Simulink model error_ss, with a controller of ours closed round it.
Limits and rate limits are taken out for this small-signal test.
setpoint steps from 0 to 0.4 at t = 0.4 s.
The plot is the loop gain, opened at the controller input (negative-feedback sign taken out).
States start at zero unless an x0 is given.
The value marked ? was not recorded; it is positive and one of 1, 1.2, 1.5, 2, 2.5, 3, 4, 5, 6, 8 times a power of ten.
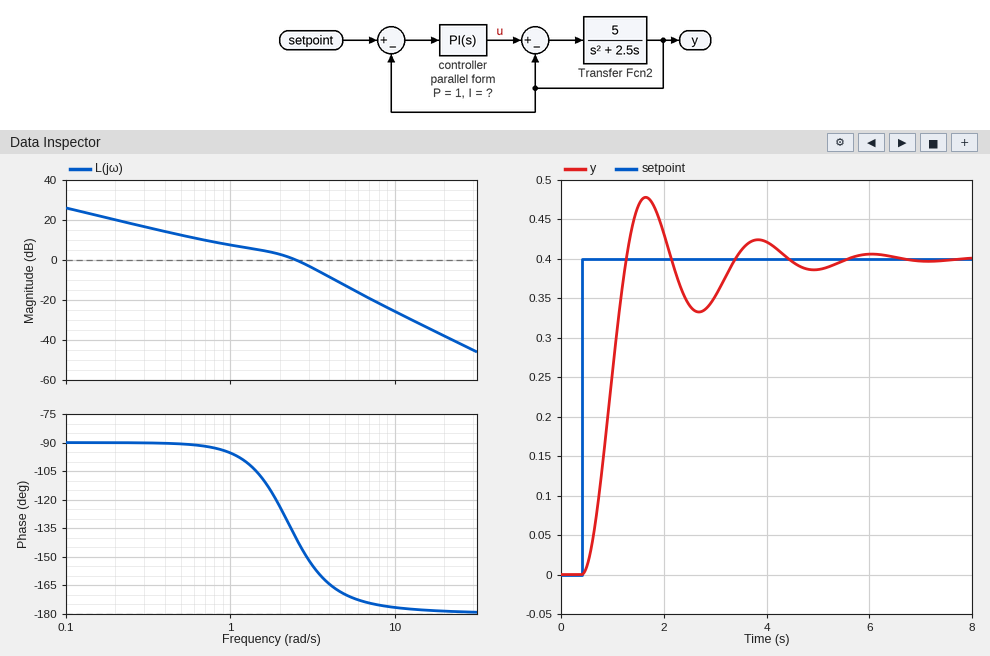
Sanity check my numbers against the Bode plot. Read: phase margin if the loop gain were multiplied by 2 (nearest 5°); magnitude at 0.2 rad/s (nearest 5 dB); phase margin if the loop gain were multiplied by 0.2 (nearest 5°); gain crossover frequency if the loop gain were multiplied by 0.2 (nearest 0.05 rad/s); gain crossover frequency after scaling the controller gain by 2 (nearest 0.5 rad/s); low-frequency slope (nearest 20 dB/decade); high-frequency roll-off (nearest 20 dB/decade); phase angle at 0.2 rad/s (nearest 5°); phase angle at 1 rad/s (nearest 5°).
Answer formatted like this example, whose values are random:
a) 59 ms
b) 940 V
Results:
a) 20°
b) 20 dB
c) 90°
d) 0.40 rad/s
e) 3.5 rad/s
f) -20 dB/decade
g) -40 dB/decade
h) -90°
i) -95°
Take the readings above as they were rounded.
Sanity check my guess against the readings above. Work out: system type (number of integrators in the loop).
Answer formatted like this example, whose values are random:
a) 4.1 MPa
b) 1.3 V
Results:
a) 1
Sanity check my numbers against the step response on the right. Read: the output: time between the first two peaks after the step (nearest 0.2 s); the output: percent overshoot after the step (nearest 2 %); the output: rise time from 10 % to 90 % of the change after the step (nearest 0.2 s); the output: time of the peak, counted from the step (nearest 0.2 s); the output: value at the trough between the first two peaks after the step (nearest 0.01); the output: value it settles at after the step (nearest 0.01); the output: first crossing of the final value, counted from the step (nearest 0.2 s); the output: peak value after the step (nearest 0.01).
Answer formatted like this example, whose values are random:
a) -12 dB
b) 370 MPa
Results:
a) 2.2 s
b) 20 %
c) 0.6 s
d) 1.2 s
e) 0.33
f) 0.40
g) 0.8 s
h) 0.48
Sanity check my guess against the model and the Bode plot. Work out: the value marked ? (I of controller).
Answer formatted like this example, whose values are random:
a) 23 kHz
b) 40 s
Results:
a) 2
